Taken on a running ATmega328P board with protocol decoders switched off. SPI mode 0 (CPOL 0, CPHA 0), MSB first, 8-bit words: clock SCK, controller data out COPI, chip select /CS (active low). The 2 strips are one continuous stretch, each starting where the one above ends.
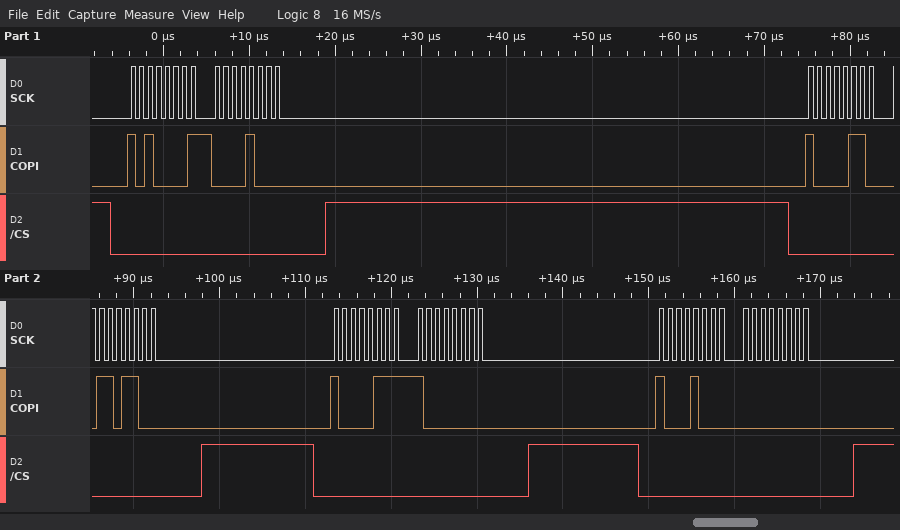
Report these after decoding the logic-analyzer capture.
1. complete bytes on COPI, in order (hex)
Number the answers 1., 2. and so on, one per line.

1. A1 08 86 6C 87 80 88 00
